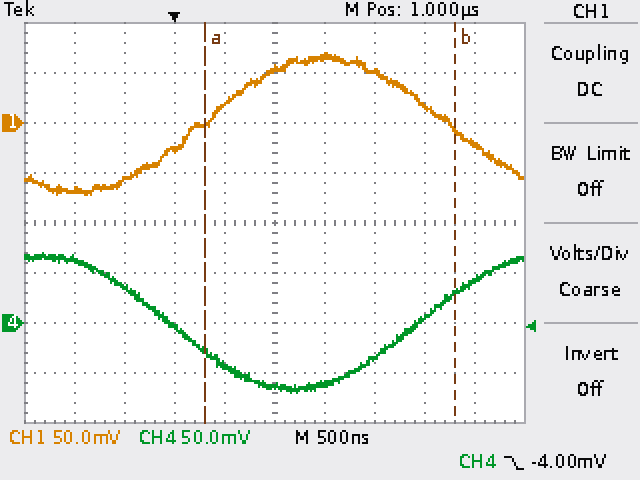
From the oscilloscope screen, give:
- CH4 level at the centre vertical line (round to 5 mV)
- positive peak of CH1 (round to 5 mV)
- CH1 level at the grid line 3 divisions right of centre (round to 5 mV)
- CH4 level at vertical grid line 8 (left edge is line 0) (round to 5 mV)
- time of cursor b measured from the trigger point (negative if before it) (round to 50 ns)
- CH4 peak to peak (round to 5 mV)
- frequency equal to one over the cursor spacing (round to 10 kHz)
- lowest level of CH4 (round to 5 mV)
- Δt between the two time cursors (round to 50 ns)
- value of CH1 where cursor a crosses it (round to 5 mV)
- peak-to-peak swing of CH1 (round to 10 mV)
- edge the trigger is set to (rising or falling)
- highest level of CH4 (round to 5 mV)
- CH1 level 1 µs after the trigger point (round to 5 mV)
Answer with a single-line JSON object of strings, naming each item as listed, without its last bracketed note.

{"CH4 level at the centre vertical line": "-65 mV", "positive peak of CH1": "70 mV", "CH1 level at the grid line 3 divisions right of centre": "15 mV", "CH4 level at vertical grid line 8 (left edge is line 0)": "5 mV", "time of cursor b measured from the trigger point (negative if before it)": "+2.80 µs", "CH4 peak to peak": "140 mV", "frequency equal to one over the cursor spacing": "400 kHz", "lowest level of CH4": "-70 mV", "Δt between the two time cursors": "2.50 µs", "value of CH1 where cursor a crosses it": "0 mV", "peak-to-peak swing of CH1": "140 mV", "edge the trigger is set to": "falling", "highest level of CH4": "70 mV", "CH1 level 1 µs after the trigger point": "55 mV"}
